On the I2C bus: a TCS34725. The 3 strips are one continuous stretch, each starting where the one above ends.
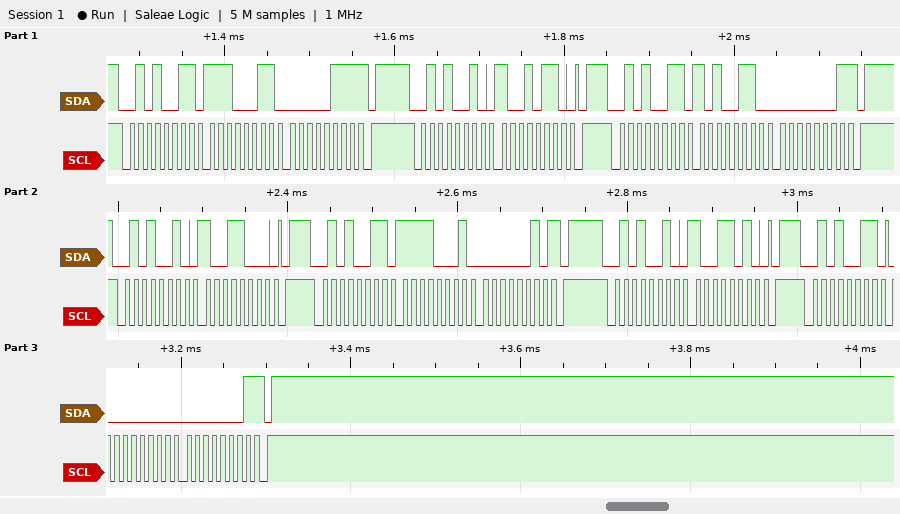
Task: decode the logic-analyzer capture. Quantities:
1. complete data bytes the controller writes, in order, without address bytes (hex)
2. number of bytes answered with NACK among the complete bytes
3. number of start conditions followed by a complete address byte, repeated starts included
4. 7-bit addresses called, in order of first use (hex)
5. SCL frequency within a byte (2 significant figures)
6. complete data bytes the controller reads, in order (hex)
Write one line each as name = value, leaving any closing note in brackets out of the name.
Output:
complete data bytes the controller writes, in order, without address bytes = 96 98 9A
number of bytes answered with NACK among the complete bytes = 4
number of start conditions followed by a complete address byte, repeated starts included = 7
7-bit addresses called, in order of first use = 0x29
SCL frequency within a byte = 100 kHz
complete data bytes the controller reads, in order = E3 07 A6 01 F1 02 00 01
